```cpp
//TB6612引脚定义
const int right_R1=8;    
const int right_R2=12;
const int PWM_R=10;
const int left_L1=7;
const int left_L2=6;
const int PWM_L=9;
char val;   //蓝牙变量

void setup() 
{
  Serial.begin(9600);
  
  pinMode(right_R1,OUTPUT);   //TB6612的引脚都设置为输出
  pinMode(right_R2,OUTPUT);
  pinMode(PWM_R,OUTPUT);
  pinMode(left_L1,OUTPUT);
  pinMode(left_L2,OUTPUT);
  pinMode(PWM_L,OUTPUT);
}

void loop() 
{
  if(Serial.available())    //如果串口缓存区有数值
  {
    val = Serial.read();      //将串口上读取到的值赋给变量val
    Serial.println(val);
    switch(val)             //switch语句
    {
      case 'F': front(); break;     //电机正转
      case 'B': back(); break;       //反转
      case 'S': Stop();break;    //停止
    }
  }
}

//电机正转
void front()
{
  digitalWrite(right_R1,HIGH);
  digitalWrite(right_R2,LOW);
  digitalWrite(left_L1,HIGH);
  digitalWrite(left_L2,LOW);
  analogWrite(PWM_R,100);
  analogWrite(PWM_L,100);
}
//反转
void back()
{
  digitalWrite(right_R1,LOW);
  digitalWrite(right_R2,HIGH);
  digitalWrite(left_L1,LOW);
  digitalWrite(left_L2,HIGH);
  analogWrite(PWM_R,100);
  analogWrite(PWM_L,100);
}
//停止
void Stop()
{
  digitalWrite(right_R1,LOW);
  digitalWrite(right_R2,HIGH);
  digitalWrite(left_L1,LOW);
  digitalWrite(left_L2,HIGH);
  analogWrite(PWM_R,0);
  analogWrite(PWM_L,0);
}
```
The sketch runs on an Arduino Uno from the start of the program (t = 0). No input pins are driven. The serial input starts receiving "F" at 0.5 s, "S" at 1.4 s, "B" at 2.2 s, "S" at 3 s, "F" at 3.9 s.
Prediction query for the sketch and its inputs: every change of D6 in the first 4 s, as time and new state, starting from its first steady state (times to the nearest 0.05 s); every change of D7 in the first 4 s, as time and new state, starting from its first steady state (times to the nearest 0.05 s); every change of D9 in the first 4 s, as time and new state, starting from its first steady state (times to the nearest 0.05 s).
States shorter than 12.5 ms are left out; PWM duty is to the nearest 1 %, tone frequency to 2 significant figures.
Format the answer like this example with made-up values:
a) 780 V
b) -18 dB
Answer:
a) 0 s low; 1.4 s high; 3.9 s low
b) 0 s low; 0.5 s high; 1.4 s low; 3.9 s high
c) 0 s low; 0.5 s PWM 39 %; 1.4 s low; 2.2 s PWM 39 %; 3 s low; 3.9 s PWM 39 %
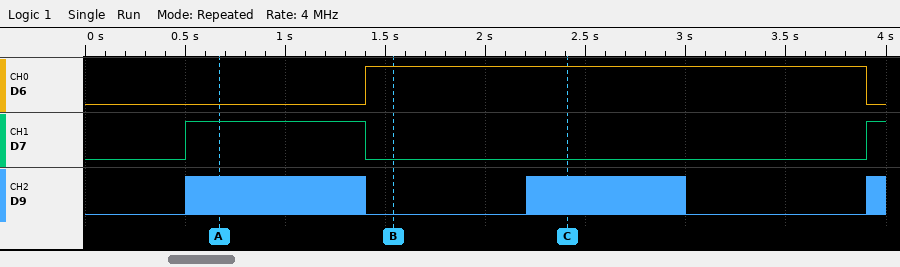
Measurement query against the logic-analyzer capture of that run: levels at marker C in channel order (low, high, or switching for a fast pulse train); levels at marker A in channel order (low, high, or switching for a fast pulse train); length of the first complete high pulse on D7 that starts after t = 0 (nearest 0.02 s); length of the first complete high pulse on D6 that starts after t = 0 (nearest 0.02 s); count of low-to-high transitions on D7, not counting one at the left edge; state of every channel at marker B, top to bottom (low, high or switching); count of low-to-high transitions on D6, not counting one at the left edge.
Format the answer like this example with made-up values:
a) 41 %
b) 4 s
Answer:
a) D6 high, D7 low, D9 switching
b) D6 low, D7 high, D9 switching
c) 0.90 s
d) 2.50 s
e) 2
f) D6 high, D7 low, D9 low
g) 1
